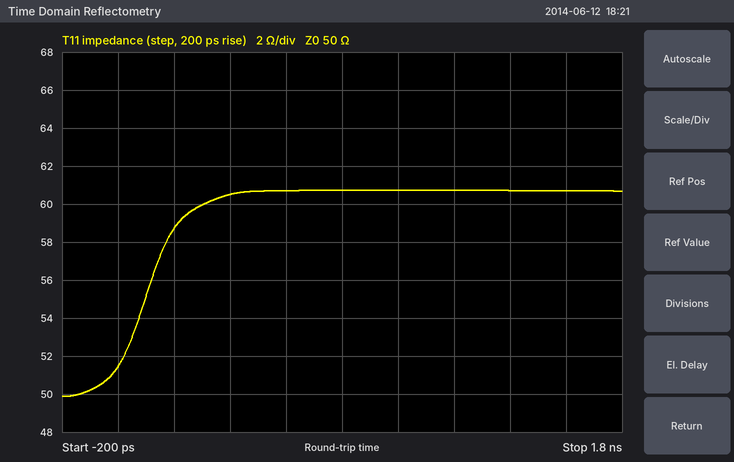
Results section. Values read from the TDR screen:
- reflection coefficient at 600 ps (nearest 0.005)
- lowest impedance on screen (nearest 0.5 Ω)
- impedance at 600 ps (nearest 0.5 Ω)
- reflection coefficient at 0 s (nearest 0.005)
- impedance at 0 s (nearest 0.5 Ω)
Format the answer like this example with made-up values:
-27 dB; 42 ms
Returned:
+0.095; 50.0 Ω; 60.5 Ω; +0.015; 51.5 Ω
